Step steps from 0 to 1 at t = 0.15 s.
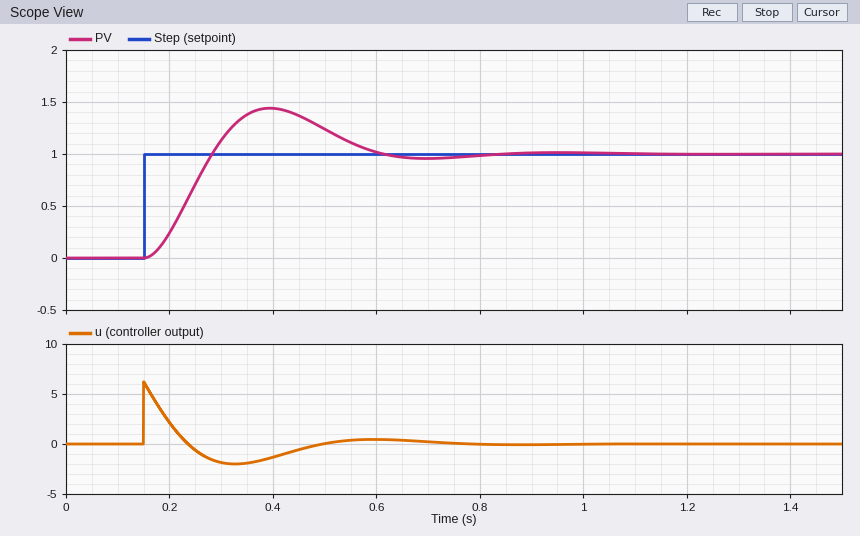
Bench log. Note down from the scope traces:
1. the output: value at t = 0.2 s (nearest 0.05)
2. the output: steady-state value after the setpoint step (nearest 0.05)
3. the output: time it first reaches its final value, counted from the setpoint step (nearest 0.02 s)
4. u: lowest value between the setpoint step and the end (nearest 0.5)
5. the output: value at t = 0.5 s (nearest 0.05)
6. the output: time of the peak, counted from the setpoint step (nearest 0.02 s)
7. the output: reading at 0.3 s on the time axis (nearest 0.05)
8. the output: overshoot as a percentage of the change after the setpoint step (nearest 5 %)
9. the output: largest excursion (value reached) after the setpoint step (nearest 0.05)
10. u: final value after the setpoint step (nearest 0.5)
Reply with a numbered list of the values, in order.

1. 0.25
2. 1.00
3. 0.14 s
4. -2.0
5. 1.25
6. 0.24 s
7. 1.15
8. 45 %
9. 1.45
10. 0.0
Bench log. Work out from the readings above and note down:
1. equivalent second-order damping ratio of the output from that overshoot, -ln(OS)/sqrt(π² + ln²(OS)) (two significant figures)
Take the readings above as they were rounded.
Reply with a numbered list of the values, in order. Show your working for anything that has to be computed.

1. ln(0.45) = -0.799; 0.799 / sqrt(9.870 + 0.638) = 0.25
